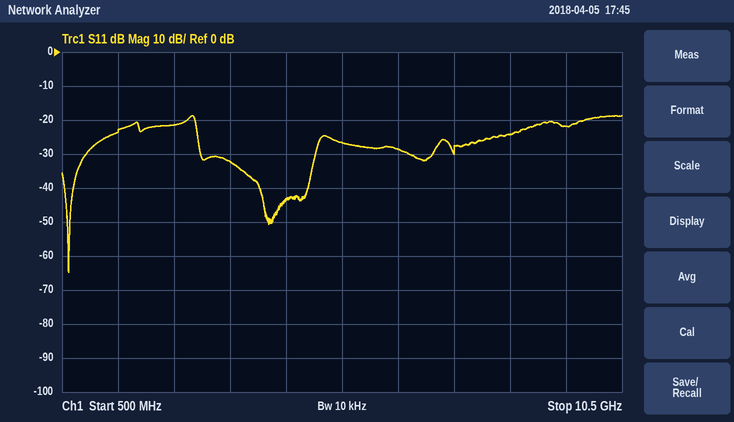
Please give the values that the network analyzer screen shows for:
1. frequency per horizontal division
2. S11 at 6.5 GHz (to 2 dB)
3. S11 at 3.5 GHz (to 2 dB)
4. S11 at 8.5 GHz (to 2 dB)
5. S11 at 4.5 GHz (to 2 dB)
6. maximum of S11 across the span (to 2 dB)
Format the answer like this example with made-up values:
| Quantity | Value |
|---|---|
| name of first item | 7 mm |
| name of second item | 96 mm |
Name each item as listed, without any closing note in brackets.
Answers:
| Quantity | Value |
|---|---|
| frequency per horizontal division | 1 GHz |
| S11 at 6.5 GHz | -28 dB |
| S11 at 3.5 GHz | -32 dB |
| S11 at 8.5 GHz | -24 dB |
| S11 at 4.5 GHz | -44 dB |
| maximum of S11 across the span | -18 dB |
